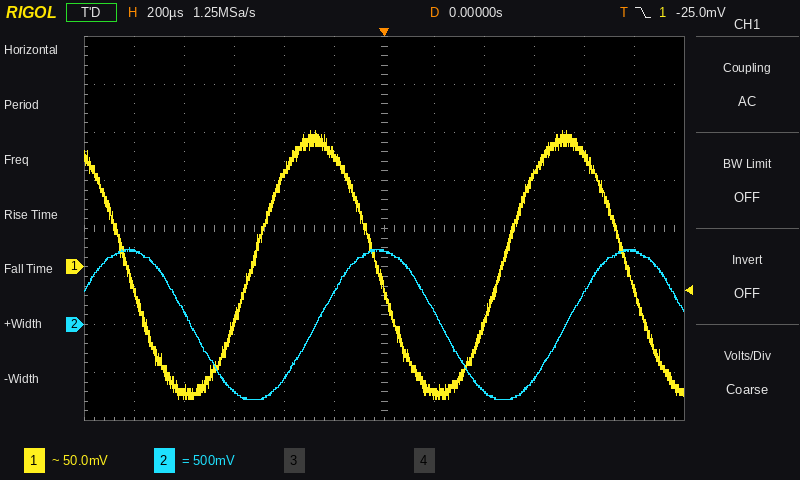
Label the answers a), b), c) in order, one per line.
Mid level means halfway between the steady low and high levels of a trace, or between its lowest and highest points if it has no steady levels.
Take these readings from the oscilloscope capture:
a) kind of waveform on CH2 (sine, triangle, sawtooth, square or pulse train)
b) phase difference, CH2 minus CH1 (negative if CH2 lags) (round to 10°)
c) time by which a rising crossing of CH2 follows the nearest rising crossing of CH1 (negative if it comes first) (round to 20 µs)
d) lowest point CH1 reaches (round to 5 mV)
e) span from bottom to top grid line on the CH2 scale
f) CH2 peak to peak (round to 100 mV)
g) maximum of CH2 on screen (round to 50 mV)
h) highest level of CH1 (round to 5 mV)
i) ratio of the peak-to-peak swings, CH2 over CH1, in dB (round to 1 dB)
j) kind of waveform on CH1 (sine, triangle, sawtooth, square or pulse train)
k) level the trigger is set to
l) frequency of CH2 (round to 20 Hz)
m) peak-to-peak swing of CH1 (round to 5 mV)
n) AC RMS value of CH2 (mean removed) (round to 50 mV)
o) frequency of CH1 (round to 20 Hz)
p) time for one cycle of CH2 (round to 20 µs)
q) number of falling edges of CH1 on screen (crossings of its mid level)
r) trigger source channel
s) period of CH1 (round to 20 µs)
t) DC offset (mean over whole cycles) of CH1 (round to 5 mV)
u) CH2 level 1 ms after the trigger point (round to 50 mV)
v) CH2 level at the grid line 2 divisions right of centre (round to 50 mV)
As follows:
a) sine
b) -90°
c) +260 µs
d) -140 mV
e) 4 V
f) 1.60 V
g) 800 mV
h) 140 mV
i) 15 dB
j) sine
k) -25.0 mV
l) 1.00 kHz
m) 280 mV
n) 550 mV
o) 1.00 kHz
p) 1.00 ms
q) 3
r) CH1
s) 1.00 ms
t) 0 mV
u) 750 mV
v) -700 mV
